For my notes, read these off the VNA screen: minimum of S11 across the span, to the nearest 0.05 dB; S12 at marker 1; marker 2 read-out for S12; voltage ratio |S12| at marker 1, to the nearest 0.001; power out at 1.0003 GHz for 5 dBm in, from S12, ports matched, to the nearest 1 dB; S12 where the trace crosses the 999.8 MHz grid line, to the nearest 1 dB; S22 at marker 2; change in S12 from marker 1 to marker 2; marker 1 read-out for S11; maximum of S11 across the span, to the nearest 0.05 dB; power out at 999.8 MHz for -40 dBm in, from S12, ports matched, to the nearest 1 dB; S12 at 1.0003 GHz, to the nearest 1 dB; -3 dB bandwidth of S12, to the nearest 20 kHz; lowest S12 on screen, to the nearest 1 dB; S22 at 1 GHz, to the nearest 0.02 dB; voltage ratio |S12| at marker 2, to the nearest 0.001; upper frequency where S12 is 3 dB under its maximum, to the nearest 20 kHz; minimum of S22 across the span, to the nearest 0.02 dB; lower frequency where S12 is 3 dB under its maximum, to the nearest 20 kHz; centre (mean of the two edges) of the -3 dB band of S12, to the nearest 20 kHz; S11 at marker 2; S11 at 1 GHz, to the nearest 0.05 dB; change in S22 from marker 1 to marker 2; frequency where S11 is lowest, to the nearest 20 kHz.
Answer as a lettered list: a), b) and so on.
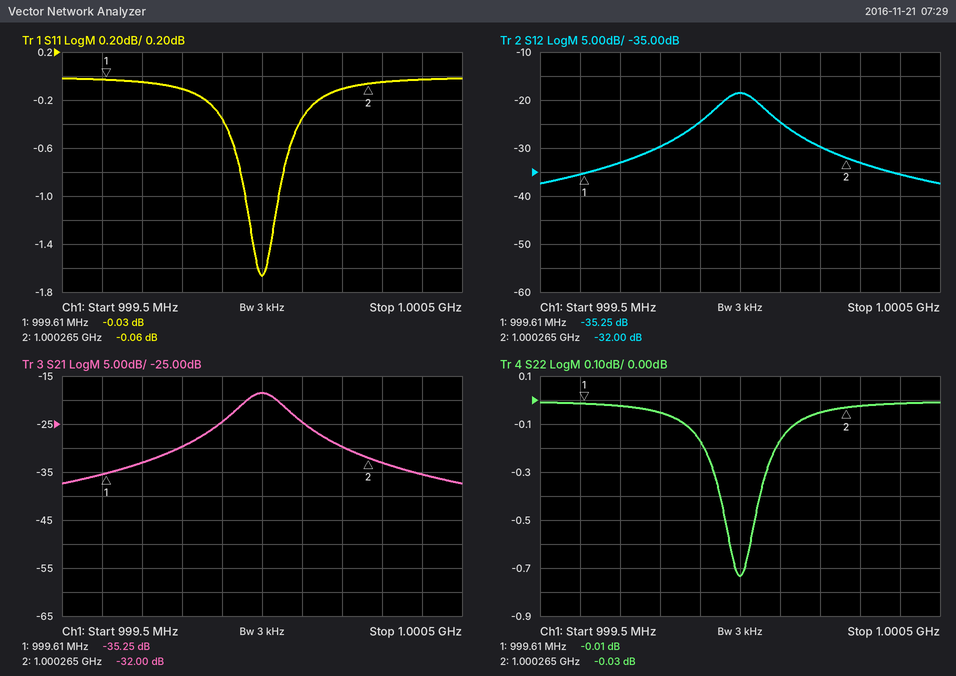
a) -1.65 dB
b) -35.25 dB
c) -32.00 dB
d) 0.017
e) -28 dBm
f) -30 dB
g) -0.03 dB
h) 3.25 dB
i) -0.03 dB
j) 0.00 dB
k) -70 dBm
l) -33 dB
m) 120 kHz
n) -37 dB
o) -0.74 dB
p) 0.025
q) 1.00006 GHz
r) -0.74 dB
s) 999.94 MHz
t) 1.00000 GHz
u) -0.06 dB
v) -1.65 dB
w) -0.02 dB
x) 1.00000 GHz
